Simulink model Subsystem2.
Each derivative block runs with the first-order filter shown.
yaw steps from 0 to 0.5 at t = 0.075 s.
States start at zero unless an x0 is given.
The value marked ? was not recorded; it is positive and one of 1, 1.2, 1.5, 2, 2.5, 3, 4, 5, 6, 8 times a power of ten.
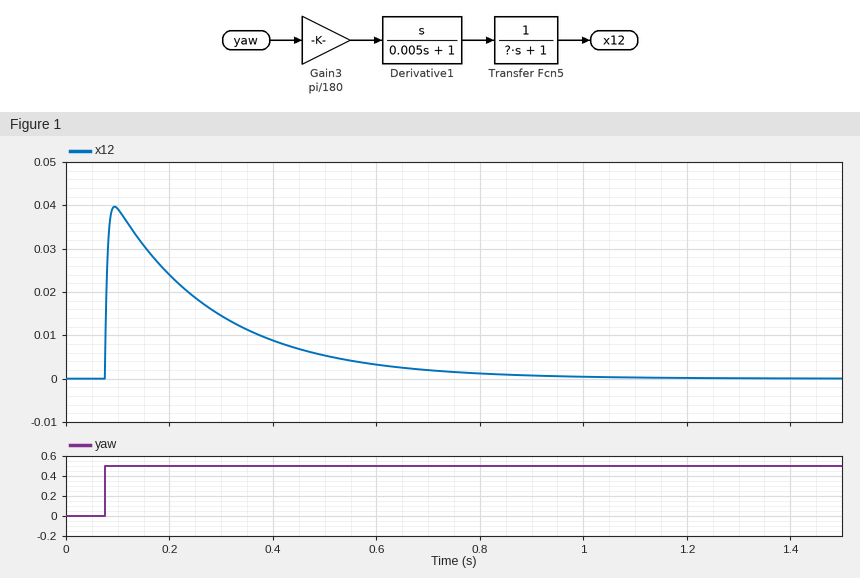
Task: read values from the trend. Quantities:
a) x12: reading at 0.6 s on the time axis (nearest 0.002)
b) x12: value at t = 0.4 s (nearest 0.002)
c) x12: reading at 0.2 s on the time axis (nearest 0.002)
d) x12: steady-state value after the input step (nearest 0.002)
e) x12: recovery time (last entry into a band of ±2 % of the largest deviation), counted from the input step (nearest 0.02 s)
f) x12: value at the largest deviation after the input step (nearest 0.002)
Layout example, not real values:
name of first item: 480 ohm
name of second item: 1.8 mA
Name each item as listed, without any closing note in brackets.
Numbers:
x12: reading at 0.6 s on the time axis: 0.004
x12: value at t = 0.4 s: 0.008
x12: reading at 0.2 s on the time axis: 0.024
x12: steady-state value after the input step: 0.000
x12: recovery time (last entry into a band of ±2 % of the largest deviation), counted from the input step: 0.80 s
x12: value at the largest deviation after the input step: 0.040
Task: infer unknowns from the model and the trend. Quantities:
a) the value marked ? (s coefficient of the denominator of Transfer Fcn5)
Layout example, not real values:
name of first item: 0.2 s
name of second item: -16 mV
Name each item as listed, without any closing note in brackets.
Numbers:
the value marked ?: 0.2
